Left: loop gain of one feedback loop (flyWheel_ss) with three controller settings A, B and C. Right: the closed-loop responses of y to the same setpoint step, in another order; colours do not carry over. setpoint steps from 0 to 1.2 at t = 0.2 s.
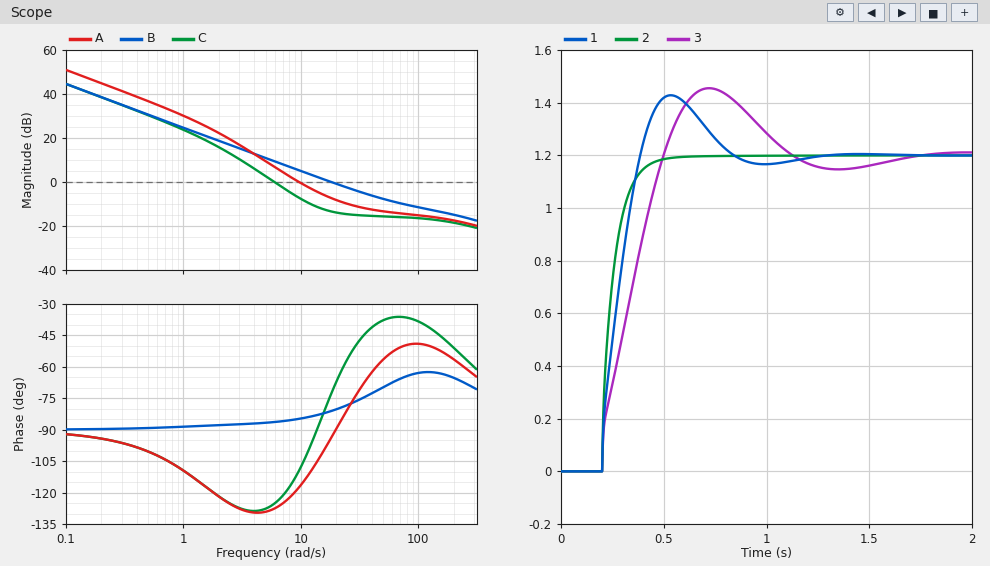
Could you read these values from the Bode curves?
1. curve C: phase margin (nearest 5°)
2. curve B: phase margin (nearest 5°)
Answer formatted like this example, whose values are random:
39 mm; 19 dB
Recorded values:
55°; 100°
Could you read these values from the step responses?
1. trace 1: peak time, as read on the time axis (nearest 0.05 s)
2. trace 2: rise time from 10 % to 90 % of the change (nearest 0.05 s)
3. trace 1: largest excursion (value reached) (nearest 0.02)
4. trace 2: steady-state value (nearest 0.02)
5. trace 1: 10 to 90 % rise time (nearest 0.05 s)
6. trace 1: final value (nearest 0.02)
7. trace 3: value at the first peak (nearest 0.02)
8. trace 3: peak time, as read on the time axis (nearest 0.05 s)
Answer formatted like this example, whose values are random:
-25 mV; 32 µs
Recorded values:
0.55 s; 0.15 s; 1.42; 1.20; 0.15 s; 1.20; 1.46; 0.70 s
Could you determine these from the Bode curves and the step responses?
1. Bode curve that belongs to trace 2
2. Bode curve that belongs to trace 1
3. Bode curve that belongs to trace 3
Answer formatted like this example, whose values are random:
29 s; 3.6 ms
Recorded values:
B; A; C
